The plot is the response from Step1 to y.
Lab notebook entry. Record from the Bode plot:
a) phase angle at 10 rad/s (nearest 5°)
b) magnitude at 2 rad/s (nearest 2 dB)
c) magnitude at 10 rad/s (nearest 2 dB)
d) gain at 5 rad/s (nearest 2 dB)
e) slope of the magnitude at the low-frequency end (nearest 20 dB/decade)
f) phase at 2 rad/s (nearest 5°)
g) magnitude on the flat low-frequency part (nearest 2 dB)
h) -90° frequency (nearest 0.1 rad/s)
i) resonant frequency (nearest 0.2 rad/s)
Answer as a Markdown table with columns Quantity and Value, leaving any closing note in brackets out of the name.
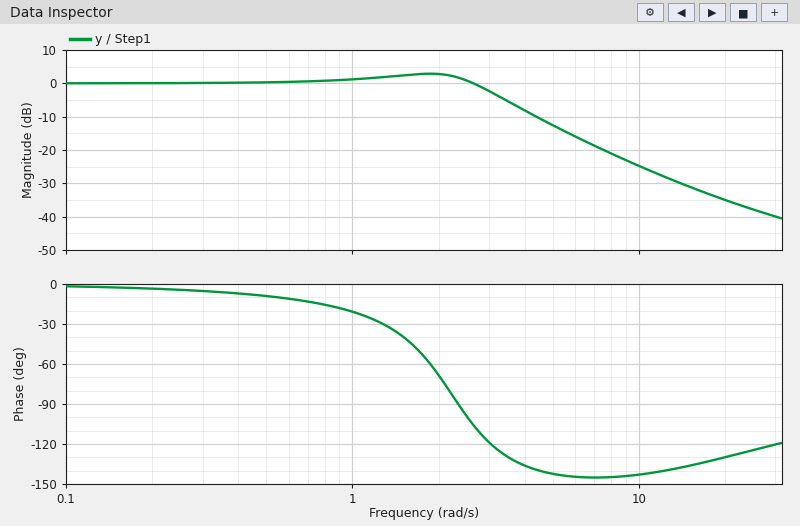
| Quantity | Value |
|---|---|
| phase angle at 10 rad/s | -145° |
| magnitude at 2 rad/s | 2 dB |
| magnitude at 10 rad/s | -24 dB |
| gain at 5 rad/s | -12 dB |
| slope of the magnitude at the low-frequency end | 0 dB/decade |
| phase at 2 rad/s | -70° |
| magnitude on the flat low-frequency part | 0 dB |
| -90° frequency | 2.3 rad/s |
| resonant frequency | 1.8 rad/s |
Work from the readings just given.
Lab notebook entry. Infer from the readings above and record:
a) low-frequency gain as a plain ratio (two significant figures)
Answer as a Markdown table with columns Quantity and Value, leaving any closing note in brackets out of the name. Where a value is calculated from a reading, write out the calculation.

| Quantity | Value |
|---|---|
| low-frequency gain as a plain ratio | 10^(0 / 20) = 1.0 |
